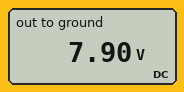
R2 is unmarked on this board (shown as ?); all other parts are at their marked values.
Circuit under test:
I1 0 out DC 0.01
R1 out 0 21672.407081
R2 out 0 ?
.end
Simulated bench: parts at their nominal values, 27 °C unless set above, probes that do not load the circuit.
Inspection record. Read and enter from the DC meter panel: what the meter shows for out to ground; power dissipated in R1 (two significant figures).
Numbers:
7.90 V
2.9 mW
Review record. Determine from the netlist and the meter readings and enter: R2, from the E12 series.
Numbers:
820 Ω
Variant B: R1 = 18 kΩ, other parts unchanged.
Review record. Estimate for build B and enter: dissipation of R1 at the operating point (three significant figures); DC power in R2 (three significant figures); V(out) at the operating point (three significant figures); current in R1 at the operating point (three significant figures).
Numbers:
3.42 mW
75.0 mW
7.84 V
436 µA
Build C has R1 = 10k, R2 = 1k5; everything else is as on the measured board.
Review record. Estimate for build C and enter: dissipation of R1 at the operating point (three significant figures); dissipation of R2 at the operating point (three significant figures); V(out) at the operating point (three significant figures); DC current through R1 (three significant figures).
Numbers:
17.0 mW
113 mW
13.0 V
1.30 mA
